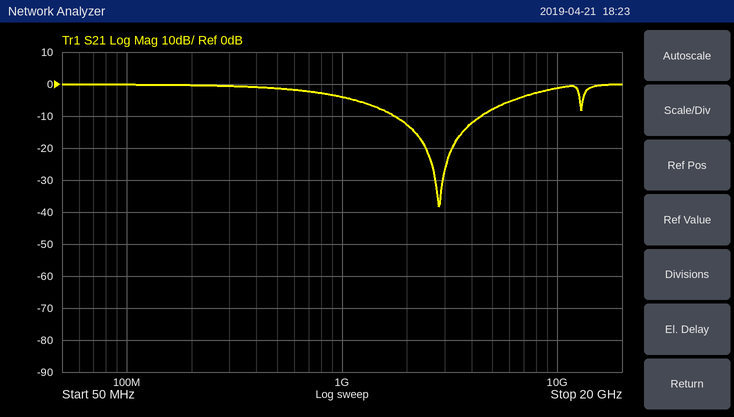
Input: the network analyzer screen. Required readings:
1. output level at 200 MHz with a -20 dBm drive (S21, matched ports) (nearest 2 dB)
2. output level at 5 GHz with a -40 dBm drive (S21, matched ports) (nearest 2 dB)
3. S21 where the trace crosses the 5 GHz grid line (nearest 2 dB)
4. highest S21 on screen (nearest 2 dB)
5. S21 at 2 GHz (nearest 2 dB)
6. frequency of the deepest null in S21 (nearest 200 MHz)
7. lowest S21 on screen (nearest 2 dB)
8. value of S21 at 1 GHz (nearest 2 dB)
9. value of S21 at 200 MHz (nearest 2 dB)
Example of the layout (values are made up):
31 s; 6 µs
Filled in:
-20 dBm; -48 dBm; -8 dB; 0 dB; -12 dB; 2.8 GHz; -38 dB; -4 dB; 0 dB
